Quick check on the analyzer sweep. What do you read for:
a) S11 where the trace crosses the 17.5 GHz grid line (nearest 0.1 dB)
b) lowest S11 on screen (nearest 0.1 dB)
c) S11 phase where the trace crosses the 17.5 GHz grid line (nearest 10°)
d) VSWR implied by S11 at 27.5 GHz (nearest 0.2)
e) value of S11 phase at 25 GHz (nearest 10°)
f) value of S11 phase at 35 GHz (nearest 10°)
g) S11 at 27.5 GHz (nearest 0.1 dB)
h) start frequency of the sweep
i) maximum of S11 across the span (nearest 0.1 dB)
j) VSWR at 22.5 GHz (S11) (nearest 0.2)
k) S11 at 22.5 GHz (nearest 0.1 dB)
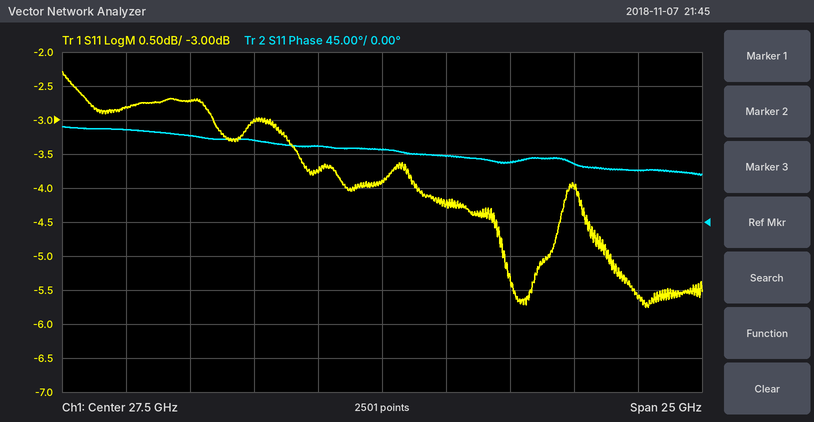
-2.8 dB
-5.8 dB
120°
4.6
100°
80°
-3.9 dB
15 GHz
-2.3 dB
5.8
-3.0 dB
